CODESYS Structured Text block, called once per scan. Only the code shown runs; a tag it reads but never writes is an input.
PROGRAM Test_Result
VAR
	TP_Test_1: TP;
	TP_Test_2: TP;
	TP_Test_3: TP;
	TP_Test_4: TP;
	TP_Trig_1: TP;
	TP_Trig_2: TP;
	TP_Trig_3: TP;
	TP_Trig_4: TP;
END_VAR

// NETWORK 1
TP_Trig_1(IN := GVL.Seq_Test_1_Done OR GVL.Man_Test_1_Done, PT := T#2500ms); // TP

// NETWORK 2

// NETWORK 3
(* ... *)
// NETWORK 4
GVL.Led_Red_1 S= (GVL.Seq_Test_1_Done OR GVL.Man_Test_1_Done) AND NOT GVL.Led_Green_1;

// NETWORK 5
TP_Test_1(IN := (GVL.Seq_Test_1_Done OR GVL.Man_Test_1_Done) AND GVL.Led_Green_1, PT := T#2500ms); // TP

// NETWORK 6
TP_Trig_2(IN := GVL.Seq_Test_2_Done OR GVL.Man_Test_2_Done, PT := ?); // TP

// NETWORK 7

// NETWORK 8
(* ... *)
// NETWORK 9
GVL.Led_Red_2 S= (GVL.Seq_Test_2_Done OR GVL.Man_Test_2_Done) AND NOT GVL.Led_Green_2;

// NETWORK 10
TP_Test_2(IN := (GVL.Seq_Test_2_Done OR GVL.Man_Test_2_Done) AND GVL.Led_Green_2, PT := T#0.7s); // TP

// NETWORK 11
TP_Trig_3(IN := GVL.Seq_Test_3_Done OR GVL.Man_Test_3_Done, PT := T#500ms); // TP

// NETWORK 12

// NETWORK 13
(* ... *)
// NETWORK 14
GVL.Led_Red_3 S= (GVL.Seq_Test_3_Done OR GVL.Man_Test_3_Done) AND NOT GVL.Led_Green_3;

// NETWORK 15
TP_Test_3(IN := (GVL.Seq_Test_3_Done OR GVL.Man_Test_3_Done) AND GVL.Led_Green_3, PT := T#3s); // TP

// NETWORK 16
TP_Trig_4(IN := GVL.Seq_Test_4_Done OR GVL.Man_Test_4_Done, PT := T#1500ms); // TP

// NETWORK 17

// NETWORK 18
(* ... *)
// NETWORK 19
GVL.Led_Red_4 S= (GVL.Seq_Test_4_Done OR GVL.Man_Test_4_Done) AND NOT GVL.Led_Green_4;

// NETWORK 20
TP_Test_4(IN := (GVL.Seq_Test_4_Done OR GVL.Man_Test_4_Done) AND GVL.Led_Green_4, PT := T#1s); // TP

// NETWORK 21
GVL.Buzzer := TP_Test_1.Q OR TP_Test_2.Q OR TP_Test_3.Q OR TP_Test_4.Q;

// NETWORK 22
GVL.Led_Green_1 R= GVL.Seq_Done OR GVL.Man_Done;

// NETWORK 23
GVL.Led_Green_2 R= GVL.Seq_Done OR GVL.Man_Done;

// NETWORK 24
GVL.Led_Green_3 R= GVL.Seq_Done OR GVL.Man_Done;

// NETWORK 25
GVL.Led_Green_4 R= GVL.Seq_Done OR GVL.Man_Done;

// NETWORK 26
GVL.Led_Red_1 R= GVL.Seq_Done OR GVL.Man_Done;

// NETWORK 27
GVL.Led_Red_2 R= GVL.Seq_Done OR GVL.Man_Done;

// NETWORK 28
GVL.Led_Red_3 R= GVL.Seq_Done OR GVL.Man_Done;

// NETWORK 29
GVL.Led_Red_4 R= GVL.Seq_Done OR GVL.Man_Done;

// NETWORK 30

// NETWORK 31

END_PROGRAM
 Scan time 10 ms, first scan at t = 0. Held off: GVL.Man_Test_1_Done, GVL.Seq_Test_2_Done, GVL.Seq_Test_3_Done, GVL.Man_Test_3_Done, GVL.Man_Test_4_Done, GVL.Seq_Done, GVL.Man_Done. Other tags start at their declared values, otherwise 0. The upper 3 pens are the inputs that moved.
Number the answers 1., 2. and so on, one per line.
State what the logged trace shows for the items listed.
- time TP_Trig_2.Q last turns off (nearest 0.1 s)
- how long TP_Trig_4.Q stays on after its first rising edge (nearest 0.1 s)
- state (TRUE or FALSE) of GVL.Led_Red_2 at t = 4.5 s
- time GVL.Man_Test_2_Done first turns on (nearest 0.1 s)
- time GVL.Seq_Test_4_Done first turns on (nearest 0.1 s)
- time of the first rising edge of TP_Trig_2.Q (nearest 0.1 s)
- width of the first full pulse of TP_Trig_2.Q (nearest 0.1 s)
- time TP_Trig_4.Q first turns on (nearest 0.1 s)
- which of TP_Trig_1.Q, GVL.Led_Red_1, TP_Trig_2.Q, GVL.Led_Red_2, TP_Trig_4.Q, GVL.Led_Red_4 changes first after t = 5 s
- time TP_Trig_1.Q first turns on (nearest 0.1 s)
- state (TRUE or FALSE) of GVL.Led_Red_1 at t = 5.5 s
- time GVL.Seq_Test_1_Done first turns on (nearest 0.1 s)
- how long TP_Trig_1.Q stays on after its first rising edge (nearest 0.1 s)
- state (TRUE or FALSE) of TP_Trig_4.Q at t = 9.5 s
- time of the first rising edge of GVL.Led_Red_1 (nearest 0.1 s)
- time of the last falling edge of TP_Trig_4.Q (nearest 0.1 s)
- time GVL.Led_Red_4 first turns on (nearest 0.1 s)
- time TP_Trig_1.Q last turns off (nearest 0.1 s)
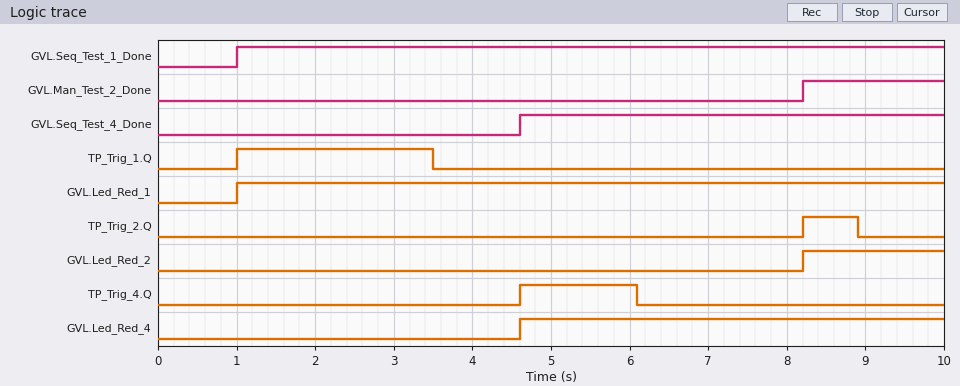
1. 8.9 s
2. 1.5 s
3. FALSE
4. 8.2 s
5. 4.6 s
6. 8.2 s
7. 0.7 s
8. 4.6 s
9. TP_Trig_4.Q
10. 1.0 s
11. TRUE
12. 1.0 s
13. 2.5 s
14. FALSE
15. 1.0 s
16. 6.1 s
17. 4.6 s
18. 3.5 s
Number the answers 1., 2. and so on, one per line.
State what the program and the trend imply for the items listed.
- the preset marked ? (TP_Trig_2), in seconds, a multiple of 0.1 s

1. 0.7 s
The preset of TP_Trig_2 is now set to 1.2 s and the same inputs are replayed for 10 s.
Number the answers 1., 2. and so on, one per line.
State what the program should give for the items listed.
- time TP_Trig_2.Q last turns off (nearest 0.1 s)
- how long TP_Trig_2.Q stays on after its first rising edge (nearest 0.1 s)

1. 9.4 s
2. 1.2 s
